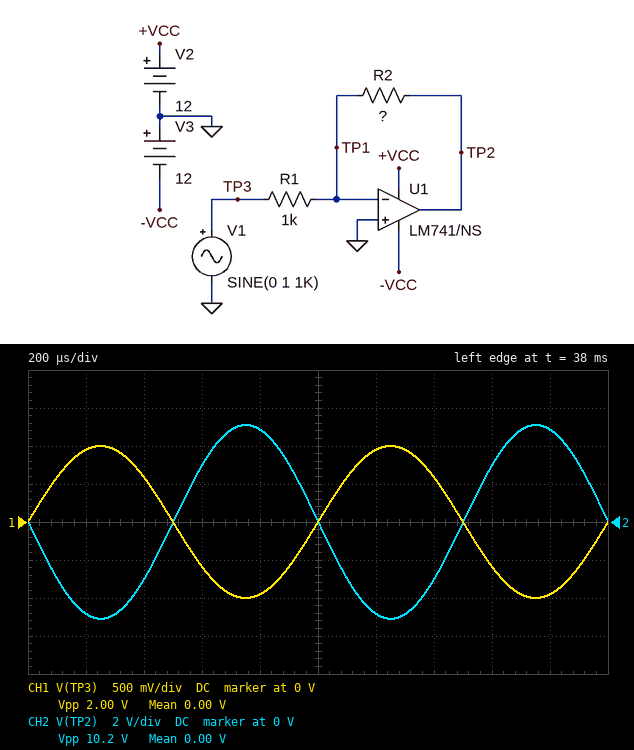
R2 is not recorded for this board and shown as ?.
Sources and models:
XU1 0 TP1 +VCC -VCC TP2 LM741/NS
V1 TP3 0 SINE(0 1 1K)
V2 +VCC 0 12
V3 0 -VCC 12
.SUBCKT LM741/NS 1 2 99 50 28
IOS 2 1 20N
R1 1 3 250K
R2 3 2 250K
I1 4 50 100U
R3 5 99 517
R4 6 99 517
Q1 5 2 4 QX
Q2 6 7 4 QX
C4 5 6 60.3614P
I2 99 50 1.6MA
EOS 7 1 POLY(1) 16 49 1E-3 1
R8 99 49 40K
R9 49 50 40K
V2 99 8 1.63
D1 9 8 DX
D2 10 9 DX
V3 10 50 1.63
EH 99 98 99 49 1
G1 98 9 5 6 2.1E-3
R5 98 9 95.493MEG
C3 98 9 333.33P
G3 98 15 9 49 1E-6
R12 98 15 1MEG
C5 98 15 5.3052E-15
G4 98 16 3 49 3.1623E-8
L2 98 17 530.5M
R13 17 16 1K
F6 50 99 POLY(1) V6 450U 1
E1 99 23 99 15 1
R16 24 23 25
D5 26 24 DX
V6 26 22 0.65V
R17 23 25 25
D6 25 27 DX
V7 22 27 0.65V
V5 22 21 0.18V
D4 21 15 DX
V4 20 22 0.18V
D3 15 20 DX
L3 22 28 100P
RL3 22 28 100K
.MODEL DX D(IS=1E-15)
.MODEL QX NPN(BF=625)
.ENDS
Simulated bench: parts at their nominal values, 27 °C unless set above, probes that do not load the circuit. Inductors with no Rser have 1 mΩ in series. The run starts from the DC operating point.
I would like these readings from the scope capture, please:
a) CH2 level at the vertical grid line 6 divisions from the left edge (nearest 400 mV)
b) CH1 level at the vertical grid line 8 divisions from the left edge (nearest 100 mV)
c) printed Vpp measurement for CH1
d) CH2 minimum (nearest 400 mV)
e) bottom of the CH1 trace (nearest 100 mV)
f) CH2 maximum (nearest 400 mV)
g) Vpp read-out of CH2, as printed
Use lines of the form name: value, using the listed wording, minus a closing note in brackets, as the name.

CH2 level at the vertical grid line 6 divisions from the left edge: -4.8 V
CH1 level at the vertical grid line 8 divisions from the left edge: -600 mV
printed Vpp measurement for CH1: 2.00 V
CH2 minimum: -5.2 V
bottom of the CH1 trace: -1.0 V
CH2 maximum: 5.2 V
Vpp read-out of CH2, as printed: 10.2 V
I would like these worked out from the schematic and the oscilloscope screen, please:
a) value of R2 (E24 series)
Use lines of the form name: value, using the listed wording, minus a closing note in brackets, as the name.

value of R2: 5.1 kΩ
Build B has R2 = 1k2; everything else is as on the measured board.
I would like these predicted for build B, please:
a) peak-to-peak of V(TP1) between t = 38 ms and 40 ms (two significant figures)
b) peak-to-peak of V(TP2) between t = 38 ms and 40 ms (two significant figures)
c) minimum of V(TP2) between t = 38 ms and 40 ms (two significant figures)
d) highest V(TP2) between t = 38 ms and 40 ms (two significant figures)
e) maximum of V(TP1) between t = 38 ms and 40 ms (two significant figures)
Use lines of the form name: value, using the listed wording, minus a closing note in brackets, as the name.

peak-to-peak of V(TP1) between t = 38 ms and 40 ms: 2.8 mV
peak-to-peak of V(TP2) between t = 38 ms and 40 ms: 2.4 V
minimum of V(TP2) between t = 38 ms and 40 ms: -1.2 V
highest V(TP2) between t = 38 ms and 40 ms: 1.2 V
maximum of V(TP1) between t = 38 ms and 40 ms: 2.4 mV
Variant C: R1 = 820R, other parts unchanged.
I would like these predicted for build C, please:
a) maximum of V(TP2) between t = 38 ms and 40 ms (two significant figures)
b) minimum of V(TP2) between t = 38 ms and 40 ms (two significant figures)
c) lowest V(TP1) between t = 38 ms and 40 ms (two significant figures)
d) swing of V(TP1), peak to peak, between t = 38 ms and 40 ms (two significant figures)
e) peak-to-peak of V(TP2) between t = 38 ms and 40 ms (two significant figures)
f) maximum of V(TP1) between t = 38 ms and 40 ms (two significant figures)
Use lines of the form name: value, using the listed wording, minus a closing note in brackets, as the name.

maximum of V(TP2) between t = 38 ms and 40 ms: 6.2 V
minimum of V(TP2) between t = 38 ms and 40 ms: -6.2 V
lowest V(TP1) between t = 38 ms and 40 ms: -5.5 mV
swing of V(TP1), peak to peak, between t = 38 ms and 40 ms: 13 mV
peak-to-peak of V(TP2) between t = 38 ms and 40 ms: 12 V
maximum of V(TP1) between t = 38 ms and 40 ms: 7.5 mV
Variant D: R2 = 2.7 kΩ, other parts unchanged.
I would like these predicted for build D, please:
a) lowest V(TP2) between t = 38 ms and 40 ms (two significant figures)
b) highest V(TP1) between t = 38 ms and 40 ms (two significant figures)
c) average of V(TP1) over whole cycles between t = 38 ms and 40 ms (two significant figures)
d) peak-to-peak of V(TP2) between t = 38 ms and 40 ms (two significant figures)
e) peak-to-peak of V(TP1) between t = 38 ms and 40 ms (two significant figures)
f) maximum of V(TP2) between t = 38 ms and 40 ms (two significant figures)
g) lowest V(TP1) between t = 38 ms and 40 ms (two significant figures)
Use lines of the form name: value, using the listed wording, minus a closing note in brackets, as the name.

lowest V(TP2) between t = 38 ms and 40 ms: -2.7 V
highest V(TP1) between t = 38 ms and 40 ms: 3.9 mV
average of V(TP1) over whole cycles between t = 38 ms and 40 ms: 1.0 mV
peak-to-peak of V(TP2) between t = 38 ms and 40 ms: 5.4 V
peak-to-peak of V(TP1) between t = 38 ms and 40 ms: 5.8 mV
maximum of V(TP2) between t = 38 ms and 40 ms: 2.7 V
lowest V(TP1) between t = 38 ms and 40 ms: -1.9 mV
